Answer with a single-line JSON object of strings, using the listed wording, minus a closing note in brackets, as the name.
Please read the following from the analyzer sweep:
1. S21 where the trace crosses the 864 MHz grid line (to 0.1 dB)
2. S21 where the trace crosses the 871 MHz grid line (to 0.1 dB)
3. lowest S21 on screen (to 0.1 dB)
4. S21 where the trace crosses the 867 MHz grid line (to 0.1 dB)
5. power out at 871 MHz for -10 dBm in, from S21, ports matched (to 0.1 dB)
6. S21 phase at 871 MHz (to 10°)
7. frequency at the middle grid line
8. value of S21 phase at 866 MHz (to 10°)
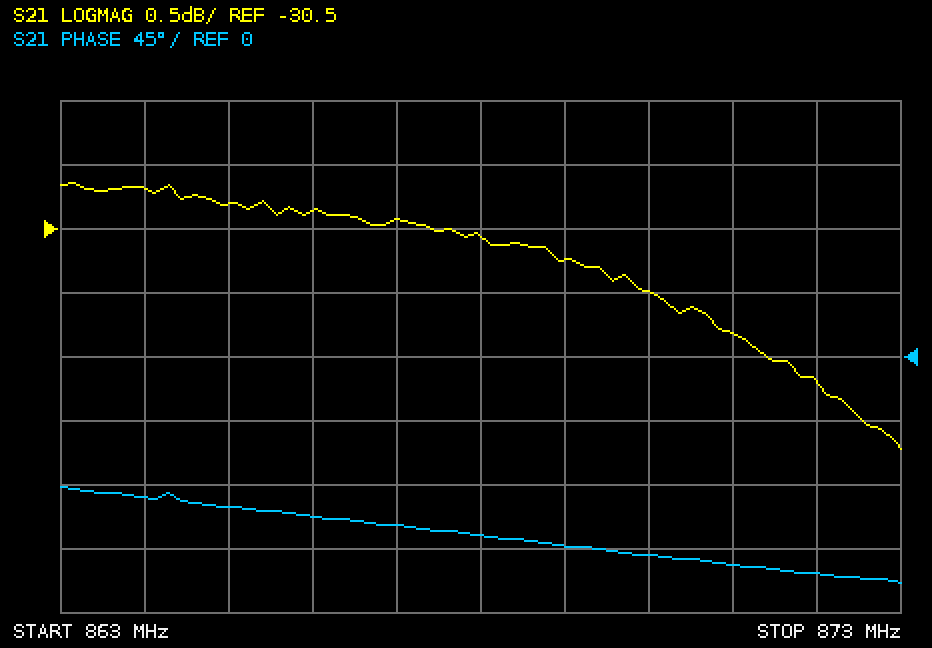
{"S21 where the trace crosses the 864 MHz grid line": "-30.2 dB", "S21 where the trace crosses the 871 MHz grid line": "-31.3 dB", "lowest S21 on screen": "-32.2 dB", "S21 where the trace crosses the 867 MHz grid line": "-30.4 dB", "power out at 871 MHz for -10 dBm in, from S21, ports matched": "-41.3 dBm", "S21 phase at 871 MHz": "-150°", "frequency at the middle grid line": "868 MHz", "value of S21 phase at 866 MHz": "-110°"}
